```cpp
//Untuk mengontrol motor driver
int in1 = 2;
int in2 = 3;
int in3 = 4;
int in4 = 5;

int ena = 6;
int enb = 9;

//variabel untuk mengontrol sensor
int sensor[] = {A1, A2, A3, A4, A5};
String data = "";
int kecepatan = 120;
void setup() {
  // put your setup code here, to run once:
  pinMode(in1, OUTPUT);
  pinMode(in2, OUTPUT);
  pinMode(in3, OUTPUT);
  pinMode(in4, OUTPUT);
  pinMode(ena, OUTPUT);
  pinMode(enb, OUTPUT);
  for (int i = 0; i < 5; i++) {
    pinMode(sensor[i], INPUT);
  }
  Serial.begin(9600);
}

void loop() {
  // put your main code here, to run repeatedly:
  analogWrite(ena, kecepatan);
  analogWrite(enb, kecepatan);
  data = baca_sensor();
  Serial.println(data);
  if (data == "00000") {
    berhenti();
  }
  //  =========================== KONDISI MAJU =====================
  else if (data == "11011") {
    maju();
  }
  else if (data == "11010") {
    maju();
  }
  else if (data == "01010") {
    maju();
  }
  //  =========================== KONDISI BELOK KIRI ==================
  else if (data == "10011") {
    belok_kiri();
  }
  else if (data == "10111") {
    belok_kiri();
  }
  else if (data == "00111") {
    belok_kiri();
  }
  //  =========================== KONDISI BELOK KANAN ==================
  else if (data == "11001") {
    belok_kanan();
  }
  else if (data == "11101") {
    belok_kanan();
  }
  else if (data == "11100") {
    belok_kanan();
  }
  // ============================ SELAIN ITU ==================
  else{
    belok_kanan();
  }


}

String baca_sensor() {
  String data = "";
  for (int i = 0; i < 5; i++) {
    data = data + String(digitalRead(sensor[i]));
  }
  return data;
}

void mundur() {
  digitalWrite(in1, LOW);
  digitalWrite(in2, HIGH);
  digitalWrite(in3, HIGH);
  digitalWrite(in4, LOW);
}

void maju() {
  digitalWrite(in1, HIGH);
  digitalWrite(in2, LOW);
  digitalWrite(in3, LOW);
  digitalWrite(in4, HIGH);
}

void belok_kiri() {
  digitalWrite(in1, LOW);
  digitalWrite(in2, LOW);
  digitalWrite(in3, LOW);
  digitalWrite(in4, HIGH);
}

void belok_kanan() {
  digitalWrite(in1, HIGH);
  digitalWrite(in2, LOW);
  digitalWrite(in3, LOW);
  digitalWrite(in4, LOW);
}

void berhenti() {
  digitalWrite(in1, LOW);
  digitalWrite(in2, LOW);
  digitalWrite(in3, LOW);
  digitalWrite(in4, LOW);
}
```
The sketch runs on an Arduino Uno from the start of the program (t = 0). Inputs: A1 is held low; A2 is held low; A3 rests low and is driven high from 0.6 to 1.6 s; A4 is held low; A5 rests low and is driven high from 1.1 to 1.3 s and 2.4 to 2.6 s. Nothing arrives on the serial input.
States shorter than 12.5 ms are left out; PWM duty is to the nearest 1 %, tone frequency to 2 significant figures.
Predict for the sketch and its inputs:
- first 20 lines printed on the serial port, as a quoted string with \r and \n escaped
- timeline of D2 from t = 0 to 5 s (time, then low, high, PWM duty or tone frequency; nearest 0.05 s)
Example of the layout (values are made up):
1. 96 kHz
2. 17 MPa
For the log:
1. "00000\r\n00000\r\n00000\r\n00000\r\n00000\r\n00000\r\n00000\r\n00000\r\n00000\r\n00000\r\n00000\r\n00000\r\n00000\r\n00000\r\n00000\r\n00000\r\n00000\r\n00000\r\n00000\r\n00000\r\n"
2. 0 s low; 0.6 s high; 1.6 s low; 2.4 s high; 2.6 s low
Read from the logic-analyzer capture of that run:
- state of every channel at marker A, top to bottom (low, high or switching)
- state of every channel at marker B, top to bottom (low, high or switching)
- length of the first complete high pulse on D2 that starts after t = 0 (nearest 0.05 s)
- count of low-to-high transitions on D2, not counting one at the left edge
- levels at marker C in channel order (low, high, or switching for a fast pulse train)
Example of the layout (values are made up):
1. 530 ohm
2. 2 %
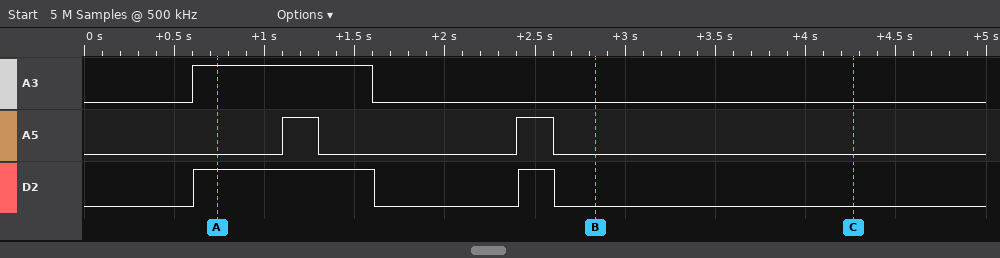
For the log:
1. A3 high, A5 low, D2 high
2. A3 low, A5 low, D2 low
3. 1.00 s
4. 2
5. A3 low, A5 low, D2 low
